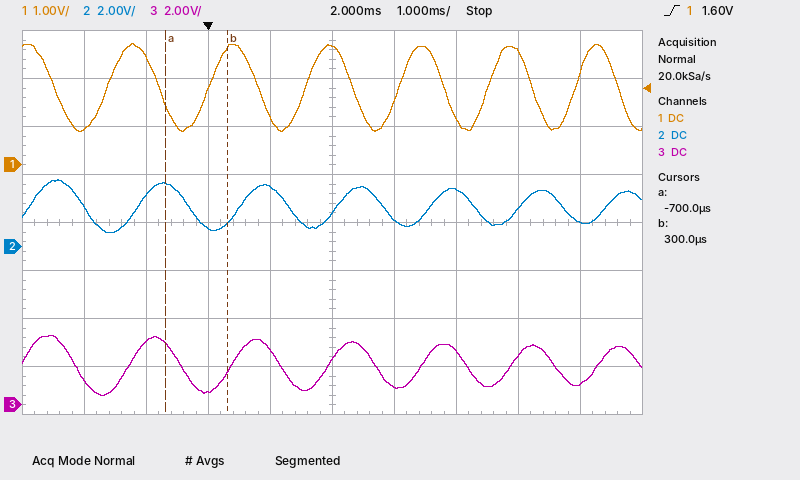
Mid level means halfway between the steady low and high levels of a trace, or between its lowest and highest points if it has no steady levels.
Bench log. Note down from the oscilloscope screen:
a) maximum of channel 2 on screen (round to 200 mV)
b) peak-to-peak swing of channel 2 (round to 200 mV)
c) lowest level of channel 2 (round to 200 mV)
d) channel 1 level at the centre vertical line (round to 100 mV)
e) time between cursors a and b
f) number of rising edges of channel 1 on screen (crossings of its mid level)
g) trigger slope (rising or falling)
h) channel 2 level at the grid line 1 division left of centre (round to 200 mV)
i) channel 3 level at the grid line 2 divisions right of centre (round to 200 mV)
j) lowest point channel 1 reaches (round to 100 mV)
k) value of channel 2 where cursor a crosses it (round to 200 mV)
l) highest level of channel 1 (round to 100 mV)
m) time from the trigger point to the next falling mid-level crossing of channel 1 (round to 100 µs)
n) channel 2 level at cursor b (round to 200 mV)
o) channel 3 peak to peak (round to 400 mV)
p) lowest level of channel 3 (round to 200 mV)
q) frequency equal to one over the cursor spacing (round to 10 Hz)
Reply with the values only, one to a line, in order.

2.8 V
2.2 V
600 mV
2.5 V
1.0 ms
6
rising
2.4 V
2.2 V
700 mV
2.6 V
2.5 V
800 µs
1.0 V
2.4 V
400 mV
1.00 kHz
